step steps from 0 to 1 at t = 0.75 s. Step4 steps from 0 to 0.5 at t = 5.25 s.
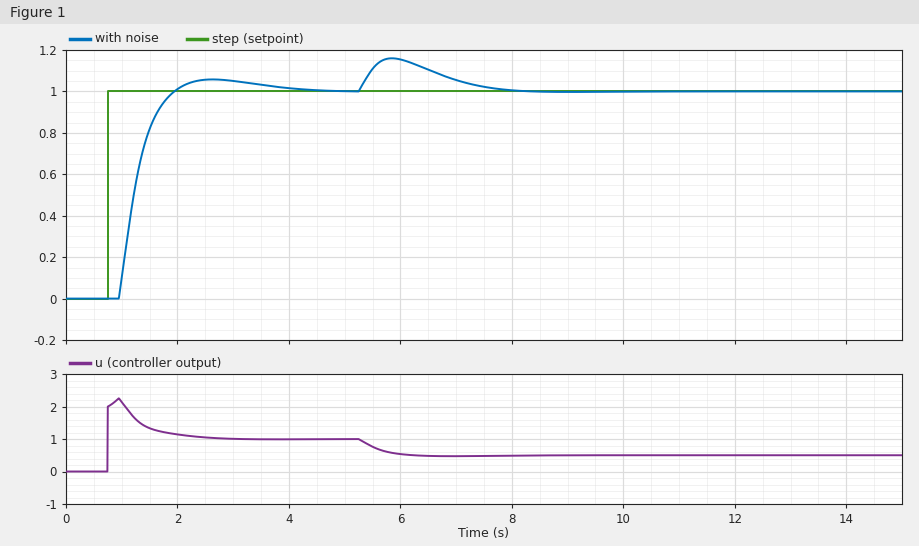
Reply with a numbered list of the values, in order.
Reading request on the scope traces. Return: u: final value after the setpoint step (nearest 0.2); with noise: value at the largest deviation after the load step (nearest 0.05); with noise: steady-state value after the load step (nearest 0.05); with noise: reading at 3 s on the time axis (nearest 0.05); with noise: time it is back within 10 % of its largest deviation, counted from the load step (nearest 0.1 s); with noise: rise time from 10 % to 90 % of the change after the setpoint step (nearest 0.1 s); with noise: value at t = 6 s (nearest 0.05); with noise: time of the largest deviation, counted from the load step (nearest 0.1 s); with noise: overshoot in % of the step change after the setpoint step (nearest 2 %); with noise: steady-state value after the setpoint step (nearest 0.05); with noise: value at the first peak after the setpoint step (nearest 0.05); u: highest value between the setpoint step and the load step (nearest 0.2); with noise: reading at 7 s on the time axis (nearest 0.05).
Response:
1. 1.0
2. 1.15
3. 1.00
4. 1.05
5. 2.4 s
6. 0.6 s
7. 1.15
8. 0.6 s
9. 6 %
10. 1.00
11. 1.05
12. 2.2
13. 1.05
